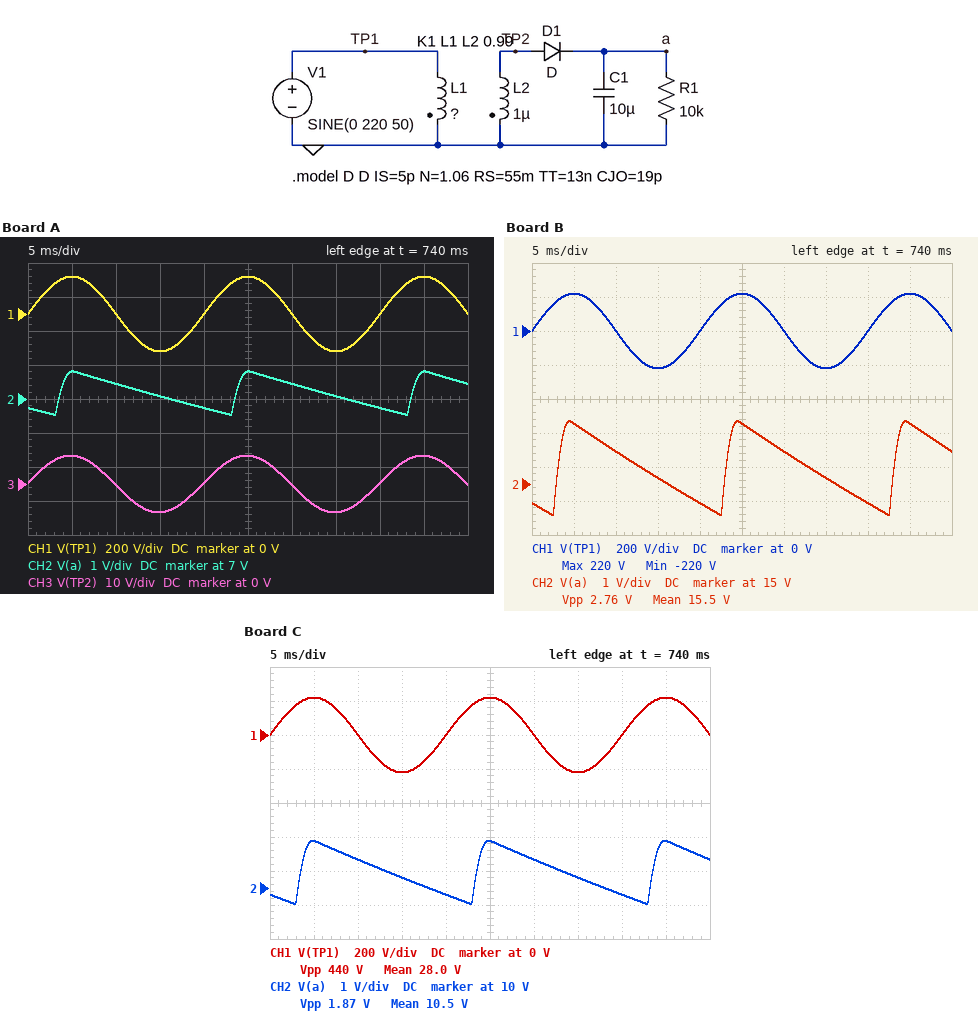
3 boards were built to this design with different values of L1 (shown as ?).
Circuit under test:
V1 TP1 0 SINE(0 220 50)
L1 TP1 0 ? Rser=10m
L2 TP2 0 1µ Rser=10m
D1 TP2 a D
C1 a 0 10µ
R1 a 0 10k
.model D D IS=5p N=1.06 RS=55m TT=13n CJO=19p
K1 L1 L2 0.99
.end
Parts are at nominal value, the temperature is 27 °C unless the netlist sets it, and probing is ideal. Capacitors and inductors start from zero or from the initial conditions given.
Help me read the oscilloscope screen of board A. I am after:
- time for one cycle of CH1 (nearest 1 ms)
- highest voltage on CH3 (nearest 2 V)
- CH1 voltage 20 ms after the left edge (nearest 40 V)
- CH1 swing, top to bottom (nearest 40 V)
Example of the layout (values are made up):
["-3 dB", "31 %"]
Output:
["20 ms", "8 V", "0 V", "440 V"]
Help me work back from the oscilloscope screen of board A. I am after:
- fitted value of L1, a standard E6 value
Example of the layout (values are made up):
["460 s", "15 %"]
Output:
["680 µH"]
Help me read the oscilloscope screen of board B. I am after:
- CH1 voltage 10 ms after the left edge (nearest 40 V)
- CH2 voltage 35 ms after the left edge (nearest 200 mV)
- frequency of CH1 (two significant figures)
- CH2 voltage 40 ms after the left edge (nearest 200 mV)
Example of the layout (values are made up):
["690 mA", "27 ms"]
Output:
["0 V", "15.2 V", "50 Hz", "14.4 V"]
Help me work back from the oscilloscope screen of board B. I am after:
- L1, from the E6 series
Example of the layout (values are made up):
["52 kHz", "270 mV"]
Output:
["150 µH"]
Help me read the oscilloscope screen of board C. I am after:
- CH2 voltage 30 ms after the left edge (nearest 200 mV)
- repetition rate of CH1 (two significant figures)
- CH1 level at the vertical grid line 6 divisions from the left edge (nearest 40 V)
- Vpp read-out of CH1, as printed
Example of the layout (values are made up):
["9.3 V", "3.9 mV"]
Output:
["10.8 V", "50 Hz", "0 V", "440 V"]
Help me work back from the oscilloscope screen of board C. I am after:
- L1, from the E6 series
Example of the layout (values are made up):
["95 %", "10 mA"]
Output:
["330 µH"]
